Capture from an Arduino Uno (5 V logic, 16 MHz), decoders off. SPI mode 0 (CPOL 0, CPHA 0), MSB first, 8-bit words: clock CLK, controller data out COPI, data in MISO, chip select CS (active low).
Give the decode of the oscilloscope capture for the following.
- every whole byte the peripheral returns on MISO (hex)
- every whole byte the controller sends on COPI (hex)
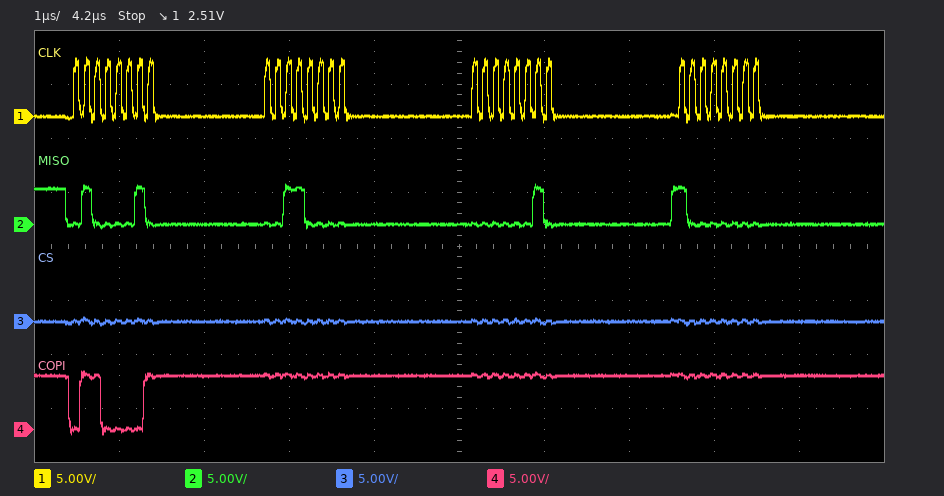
42 30 02 80
61 FF FF FF
